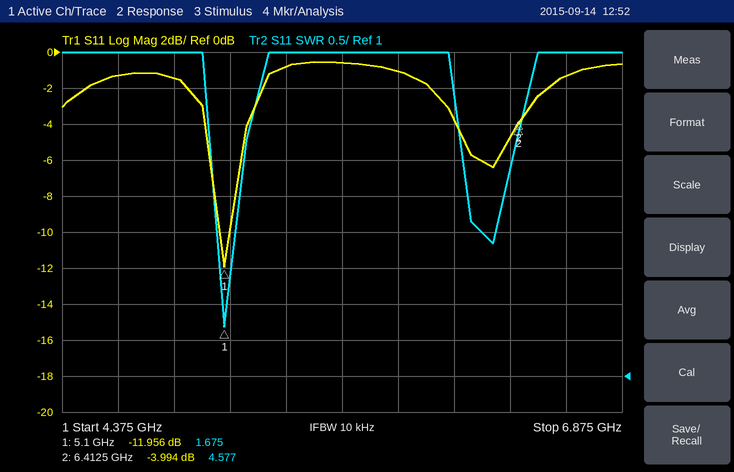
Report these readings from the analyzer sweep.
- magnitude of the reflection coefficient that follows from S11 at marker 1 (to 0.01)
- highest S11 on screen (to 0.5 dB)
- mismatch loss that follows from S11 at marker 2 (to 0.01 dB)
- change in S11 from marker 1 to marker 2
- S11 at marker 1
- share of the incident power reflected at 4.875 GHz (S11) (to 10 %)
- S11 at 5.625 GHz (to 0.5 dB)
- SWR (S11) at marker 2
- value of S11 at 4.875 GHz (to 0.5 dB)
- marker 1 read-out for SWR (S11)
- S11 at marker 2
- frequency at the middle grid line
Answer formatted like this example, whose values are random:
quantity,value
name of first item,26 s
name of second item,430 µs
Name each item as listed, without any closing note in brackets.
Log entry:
quantity,value
magnitude of the reflection coefficient that follows from S11 at marker 1,0.25
highest S11 on screen,-0.5 dB
mismatch loss that follows from S11 at marker 2,2.21 dB
change in S11 from marker 1 to marker 2,7.962 dB
S11 at marker 1,-11.956 dB
share of the incident power reflected at 4.875 GHz (S11),70 %
S11 at 5.625 GHz,-0.5 dB
SWR (S11) at marker 2,4.577
value of S11 at 4.875 GHz,-1.5 dB
marker 1 read-out for SWR,1.675
S11 at marker 2,-3.994 dB
frequency at the middle grid line,5.625 GHz
